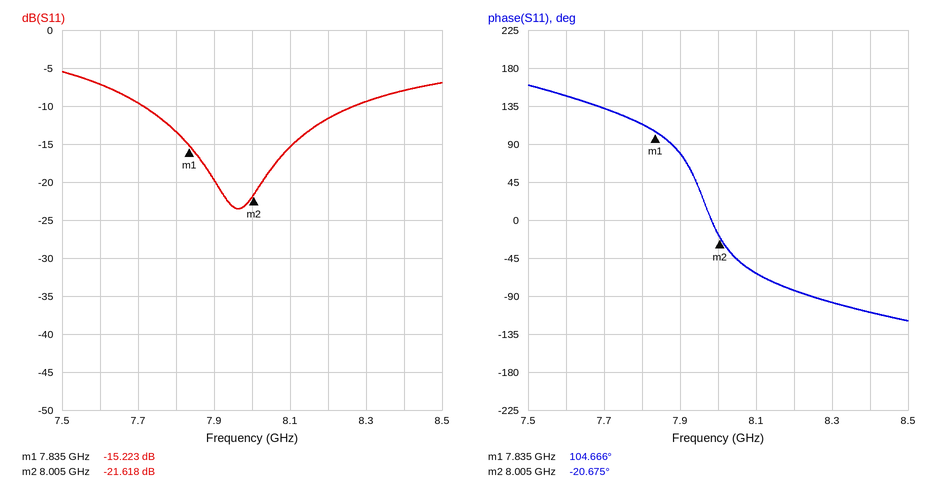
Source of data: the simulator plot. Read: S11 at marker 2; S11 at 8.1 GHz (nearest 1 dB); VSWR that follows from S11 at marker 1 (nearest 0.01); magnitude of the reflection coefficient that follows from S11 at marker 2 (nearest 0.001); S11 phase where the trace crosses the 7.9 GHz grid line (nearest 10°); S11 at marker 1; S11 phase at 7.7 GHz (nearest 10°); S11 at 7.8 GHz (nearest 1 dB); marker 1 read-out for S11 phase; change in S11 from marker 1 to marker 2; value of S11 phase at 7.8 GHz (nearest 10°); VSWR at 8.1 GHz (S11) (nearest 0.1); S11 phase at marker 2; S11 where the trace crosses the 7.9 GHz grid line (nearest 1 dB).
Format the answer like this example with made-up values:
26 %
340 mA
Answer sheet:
-21.618 dB
-15 dB
1.42
0.083
80°
-15.223 dB
130°
-13 dB
104.666°
-6.395 dB
110°
1.4
-20.675°
-20 dB
